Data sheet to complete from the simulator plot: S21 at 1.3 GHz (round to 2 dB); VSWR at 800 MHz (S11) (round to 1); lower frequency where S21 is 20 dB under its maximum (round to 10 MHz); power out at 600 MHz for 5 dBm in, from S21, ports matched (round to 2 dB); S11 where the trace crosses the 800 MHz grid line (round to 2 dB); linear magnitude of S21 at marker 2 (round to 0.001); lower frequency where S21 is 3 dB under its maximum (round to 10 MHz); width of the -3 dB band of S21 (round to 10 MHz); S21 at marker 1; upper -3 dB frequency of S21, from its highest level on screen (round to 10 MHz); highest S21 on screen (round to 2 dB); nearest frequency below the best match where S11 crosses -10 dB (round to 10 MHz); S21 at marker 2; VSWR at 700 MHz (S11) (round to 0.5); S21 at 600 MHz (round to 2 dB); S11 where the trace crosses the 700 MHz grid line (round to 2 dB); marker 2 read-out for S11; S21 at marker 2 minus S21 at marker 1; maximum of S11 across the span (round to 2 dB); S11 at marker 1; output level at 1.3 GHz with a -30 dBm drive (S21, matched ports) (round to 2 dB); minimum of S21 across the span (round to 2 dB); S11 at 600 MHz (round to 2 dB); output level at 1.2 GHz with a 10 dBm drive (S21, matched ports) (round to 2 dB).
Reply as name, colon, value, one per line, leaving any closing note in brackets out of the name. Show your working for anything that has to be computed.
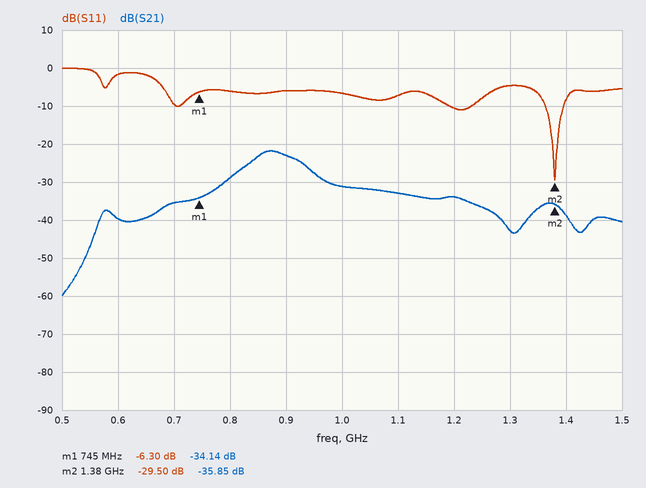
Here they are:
S21 at 1.3 GHz: -42 dB
VSWR at 800 MHz (S11): |Γ| = 10^(-6/20) = 0.5012; VSWR = (1 + 0.5012)/(1 − 0.5012) ≈ 3
lower frequency where S21 is 20 dB under its maximum: 560 MHz
power out at 600 MHz for 5 dBm in, from S21, ports matched: 5 dBm + (-40 dB) = -34 dBm
S11 where the trace crosses the 800 MHz grid line: -6 dB
linear magnitude of S21 at marker 2: 10^(-35.85/20) ≈ 0.016
lower frequency where S21 is 3 dB under its maximum: 840 MHz
width of the -3 dB band of S21: 930 MHz − 840 MHz = 90 MHz
S21 at marker 1: -34.14 dB
upper -3 dB frequency of S21, from its highest level on screen: 930 MHz
highest S21 on screen: -22 dB
nearest frequency below the best match where S11 crosses -10 dB: 1.36 GHz
S21 at marker 2: -35.85 dB
VSWR at 700 MHz (S11): |Γ| = 10^(-10/20) = 0.3162; VSWR = (1 + 0.3162)/(1 − 0.3162) ≈ 1.92, so 2.0 to the nearest 0.5
S21 at 600 MHz: -40 dB
S11 where the trace crosses the 700 MHz grid line: -10 dB
marker 2 read-out for S11: -29.50 dB
S21 at marker 2 minus S21 at marker 1: -35.85 − (-34.14) = -1.71 dB
maximum of S11 across the span: 0 dB
S11 at marker 1: -6.30 dB
output level at 1.3 GHz with a -30 dBm drive (S21, matched ports): -30 dBm + (-42 dB) = -72 dBm
minimum of S21 across the span: -60 dB
S11 at 600 MHz: -2 dB
output level at 1.2 GHz with a 10 dBm drive (S21, matched ports): 10 dBm + (-34 dB) = -24 dBm
